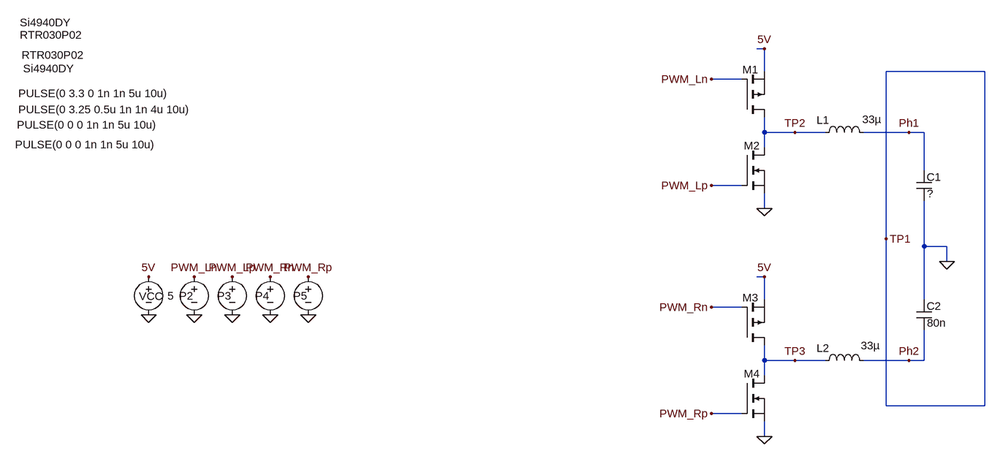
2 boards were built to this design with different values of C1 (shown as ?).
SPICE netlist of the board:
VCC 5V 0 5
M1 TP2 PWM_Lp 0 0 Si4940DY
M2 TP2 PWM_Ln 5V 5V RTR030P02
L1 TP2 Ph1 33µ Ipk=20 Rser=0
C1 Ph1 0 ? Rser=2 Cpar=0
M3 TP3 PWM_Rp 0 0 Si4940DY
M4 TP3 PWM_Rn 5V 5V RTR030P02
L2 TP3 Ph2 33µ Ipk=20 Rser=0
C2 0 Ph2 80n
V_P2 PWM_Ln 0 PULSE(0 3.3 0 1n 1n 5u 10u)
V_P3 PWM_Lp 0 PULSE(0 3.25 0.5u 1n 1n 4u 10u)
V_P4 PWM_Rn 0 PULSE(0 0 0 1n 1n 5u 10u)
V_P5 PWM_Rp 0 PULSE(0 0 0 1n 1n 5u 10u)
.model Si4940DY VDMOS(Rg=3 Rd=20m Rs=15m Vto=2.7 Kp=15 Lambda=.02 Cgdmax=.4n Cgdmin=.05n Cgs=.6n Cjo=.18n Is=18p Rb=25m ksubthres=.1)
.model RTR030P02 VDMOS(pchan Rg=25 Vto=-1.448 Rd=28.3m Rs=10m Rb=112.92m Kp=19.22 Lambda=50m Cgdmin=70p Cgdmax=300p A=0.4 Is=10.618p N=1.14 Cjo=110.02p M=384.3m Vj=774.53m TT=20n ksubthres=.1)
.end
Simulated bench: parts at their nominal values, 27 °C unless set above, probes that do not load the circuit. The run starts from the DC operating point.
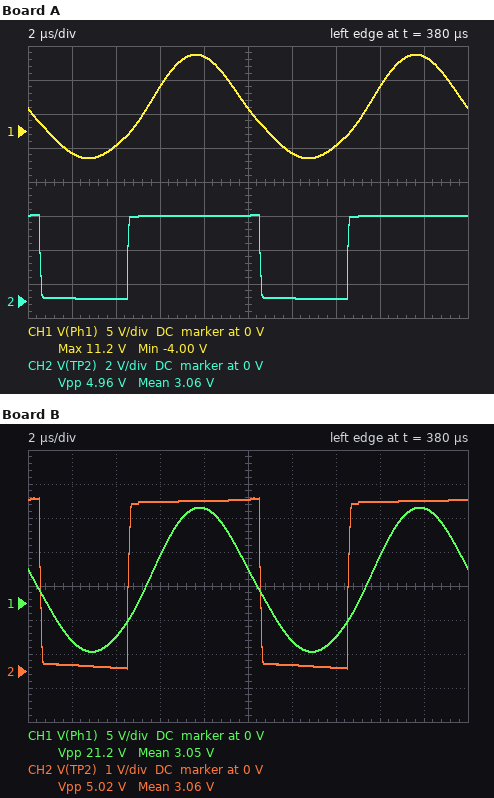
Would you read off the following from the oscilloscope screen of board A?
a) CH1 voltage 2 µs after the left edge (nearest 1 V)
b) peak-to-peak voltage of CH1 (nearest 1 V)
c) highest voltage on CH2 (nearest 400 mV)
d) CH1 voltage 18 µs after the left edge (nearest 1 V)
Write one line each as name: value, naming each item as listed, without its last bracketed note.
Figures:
CH1 voltage 2 µs after the left edge: -3 V
peak-to-peak voltage of CH1: 15 V
highest voltage on CH2: 5.2 V
CH1 voltage 18 µs after the left edge: 11 V
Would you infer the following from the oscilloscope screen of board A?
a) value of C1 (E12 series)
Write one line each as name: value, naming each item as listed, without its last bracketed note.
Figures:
value of C1: 47 nF
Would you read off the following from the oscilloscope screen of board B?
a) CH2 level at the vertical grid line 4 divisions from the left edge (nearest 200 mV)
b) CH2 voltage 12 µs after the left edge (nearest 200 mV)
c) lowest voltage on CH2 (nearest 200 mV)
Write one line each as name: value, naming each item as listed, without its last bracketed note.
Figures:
CH2 level at the vertical grid line 4 divisions from the left edge: 5.0 V
CH2 voltage 12 µs after the left edge: 200 mV
lowest voltage on CH2: 0 V
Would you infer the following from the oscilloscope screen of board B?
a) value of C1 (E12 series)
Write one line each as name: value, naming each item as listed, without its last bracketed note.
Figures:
value of C1: 56 nF
